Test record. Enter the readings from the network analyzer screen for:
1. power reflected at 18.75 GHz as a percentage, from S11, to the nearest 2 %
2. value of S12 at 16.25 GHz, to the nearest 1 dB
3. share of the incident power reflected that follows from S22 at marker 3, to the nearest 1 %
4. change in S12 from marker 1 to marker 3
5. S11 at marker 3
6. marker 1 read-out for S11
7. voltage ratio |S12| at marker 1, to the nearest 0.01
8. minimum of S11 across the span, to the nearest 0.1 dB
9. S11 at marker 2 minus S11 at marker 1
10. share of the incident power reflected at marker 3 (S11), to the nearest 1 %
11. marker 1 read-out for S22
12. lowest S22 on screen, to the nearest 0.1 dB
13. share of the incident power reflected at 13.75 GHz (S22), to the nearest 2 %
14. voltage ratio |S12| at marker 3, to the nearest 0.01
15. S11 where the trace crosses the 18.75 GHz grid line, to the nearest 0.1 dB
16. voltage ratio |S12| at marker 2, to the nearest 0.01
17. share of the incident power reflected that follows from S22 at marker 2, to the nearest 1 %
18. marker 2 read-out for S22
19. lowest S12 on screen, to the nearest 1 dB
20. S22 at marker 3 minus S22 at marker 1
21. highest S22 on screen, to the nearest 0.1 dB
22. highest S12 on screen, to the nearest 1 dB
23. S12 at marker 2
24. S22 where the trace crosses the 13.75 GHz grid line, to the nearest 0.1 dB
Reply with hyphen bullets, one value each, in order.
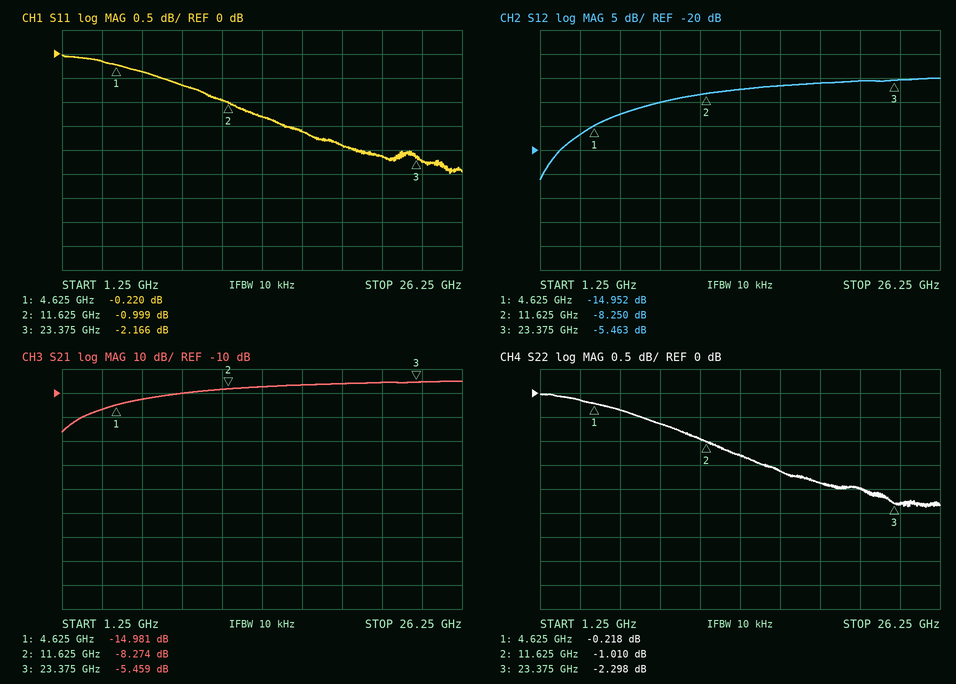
- 64 %
- -7 dB
- 59 %
- 9.489 dB
- -2.166 dB
- -0.220 dB
- 0.18
- -2.5 dB
- -0.779 dB
- 61 %
- -0.218 dB
- -2.4 dB
- 74 %
- 0.53
- -1.9 dB
- 0.39
- 79 %
- -1.010 dB
- -26 dB
- -2.080 dB
- 0.0 dB
- -5 dB
- -8.250 dB
- -1.3 dB
